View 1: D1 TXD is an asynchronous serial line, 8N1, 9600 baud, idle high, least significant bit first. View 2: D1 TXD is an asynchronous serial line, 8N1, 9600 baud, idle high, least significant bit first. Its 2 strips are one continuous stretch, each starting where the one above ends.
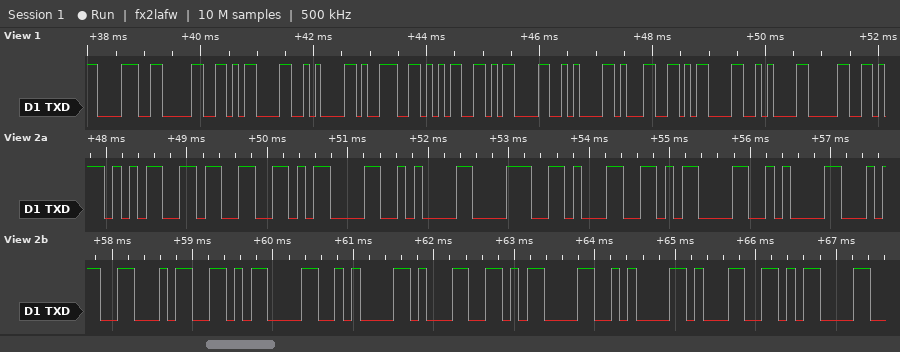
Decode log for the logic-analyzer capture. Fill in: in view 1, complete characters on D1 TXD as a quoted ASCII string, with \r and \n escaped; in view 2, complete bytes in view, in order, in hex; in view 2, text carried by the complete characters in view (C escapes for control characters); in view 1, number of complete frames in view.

"80\r\n95\r\n1\r\n0"
0x35 0x33 0x0D 0x0A 0x38 0x31 0x0D 0x0A 0x34 0x34 0x0D 0x0A 0x31 0x0D 0x0A 0x31 0x0D
"53\r\n81\r\n44\r\n1\r\n1\r"
12
